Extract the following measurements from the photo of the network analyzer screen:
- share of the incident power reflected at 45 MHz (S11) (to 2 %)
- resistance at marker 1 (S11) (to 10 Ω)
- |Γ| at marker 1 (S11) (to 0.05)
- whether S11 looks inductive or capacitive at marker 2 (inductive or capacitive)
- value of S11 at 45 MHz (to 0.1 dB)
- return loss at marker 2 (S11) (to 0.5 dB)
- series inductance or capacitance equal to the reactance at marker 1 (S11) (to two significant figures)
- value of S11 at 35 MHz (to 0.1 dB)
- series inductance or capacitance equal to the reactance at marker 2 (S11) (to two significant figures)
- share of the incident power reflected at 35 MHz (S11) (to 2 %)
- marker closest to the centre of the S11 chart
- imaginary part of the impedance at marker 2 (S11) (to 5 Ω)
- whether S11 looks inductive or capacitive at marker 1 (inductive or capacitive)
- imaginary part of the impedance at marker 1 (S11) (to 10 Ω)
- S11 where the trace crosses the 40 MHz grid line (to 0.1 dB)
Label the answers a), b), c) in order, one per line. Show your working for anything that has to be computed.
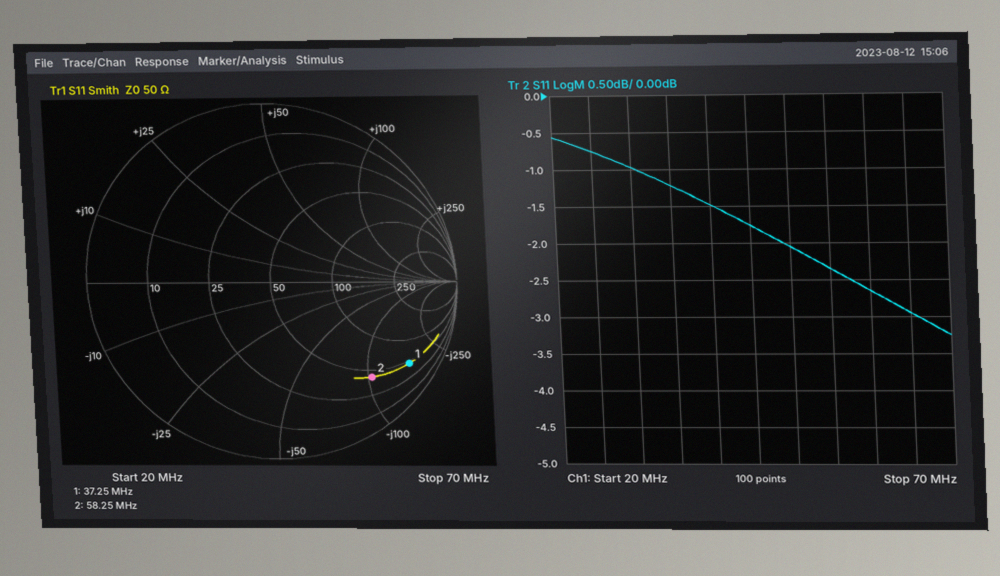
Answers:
a) 10^(-1.8/10) ≈ 66 %
b) 50 Ω
c) 0.85
d) capacitive
e) -1.8 dB
f) 2.5 dB
g) C = 1/(2π × 37.25 MHz × 160 Ω) ≈ 27 pF
h) -1.2 dB
i) C = 1/(2π × 58.25 MHz × 105 Ω) ≈ 26 pF
j) 10^(-1.2/10) ≈ 76 %
k) marker 2
l) -105 Ω
m) capacitive
n) -160 Ω
o) -1.5 dB
